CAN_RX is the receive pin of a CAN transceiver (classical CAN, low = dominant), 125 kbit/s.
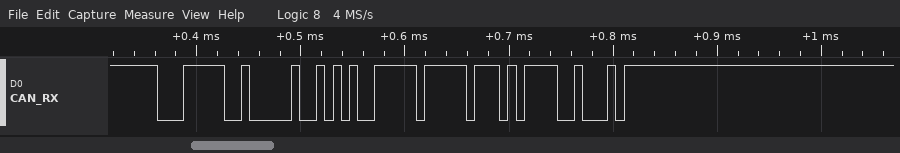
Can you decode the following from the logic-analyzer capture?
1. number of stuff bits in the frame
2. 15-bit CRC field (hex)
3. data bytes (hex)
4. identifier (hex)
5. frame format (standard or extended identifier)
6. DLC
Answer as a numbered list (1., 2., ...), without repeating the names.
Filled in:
1. 4
2. 0x6BC8
3. A7 FF
4. 0x1F4
5. standard
6. 2
